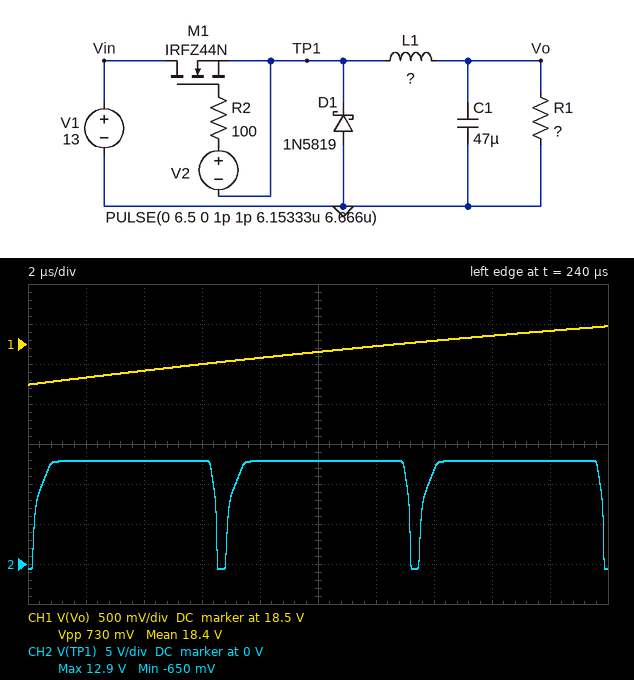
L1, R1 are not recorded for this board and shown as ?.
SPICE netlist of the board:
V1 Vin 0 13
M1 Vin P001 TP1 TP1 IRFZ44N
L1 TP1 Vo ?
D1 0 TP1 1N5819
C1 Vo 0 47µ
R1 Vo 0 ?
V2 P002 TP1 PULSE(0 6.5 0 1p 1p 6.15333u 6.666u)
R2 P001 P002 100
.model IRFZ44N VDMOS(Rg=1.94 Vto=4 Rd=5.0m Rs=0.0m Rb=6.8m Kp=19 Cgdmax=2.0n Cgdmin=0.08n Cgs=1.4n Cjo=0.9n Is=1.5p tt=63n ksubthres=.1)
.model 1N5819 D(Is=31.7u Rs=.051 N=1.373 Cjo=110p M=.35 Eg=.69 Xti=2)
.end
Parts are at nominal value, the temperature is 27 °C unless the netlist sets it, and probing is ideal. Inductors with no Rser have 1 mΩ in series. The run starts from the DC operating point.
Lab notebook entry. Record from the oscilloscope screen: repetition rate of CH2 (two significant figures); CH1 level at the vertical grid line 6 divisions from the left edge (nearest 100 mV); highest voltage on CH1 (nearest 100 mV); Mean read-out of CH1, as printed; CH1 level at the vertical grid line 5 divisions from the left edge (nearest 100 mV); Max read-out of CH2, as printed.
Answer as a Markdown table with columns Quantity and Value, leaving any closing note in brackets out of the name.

| Quantity | Value |
|---|---|
| repetition rate of CH2 | 150 kHz |
| CH1 level at the vertical grid line 6 divisions from the left edge | 18.5 V |
| highest voltage on CH1 | 18.7 V |
| Mean read-out of CH1, as printed | 18.4 V |
| CH1 level at the vertical grid line 5 divisions from the left edge | 18.4 V |
| Max read-out of CH2, as printed | 12.9 V |
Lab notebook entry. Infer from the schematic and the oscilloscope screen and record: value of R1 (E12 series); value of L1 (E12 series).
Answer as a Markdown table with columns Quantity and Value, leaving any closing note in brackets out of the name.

| Quantity | Value |
|---|---|
| value of R1 | 6.8 Ω |
| value of L1 | 180 µH |
